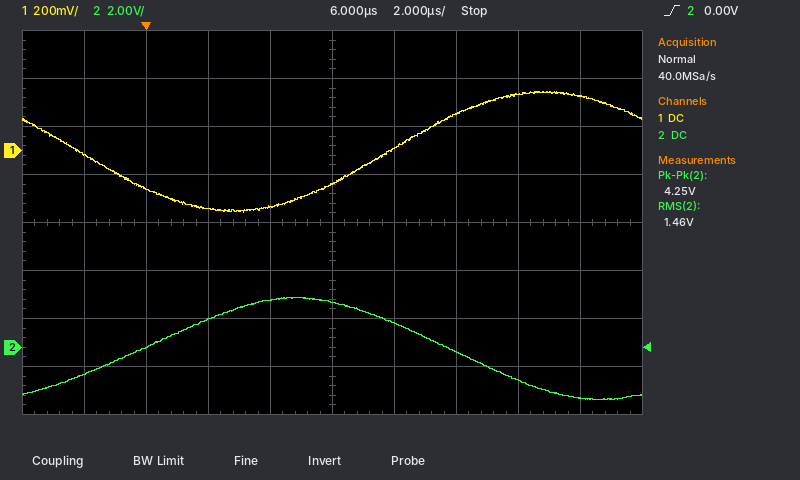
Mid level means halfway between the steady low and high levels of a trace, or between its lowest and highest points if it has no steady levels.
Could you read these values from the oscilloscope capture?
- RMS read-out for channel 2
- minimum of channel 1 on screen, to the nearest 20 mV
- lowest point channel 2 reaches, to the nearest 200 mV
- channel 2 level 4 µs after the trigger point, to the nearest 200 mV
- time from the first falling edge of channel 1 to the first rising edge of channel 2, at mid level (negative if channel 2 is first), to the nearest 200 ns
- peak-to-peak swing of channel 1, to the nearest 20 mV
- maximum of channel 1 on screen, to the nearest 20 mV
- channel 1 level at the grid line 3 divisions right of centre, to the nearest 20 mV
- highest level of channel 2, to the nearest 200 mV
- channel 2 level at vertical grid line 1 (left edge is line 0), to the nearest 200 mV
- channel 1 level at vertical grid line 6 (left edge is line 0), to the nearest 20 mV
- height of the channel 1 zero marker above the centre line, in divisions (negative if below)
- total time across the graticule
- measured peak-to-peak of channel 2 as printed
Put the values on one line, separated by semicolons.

1.46 V; -260 mV; -2.2 V; 2.0 V; +2.0 µs; 500 mV; 240 mV; 240 mV; 2.0 V; -1.2 V; 0 mV; +1.5 div; 20 µs; 4.25 V
